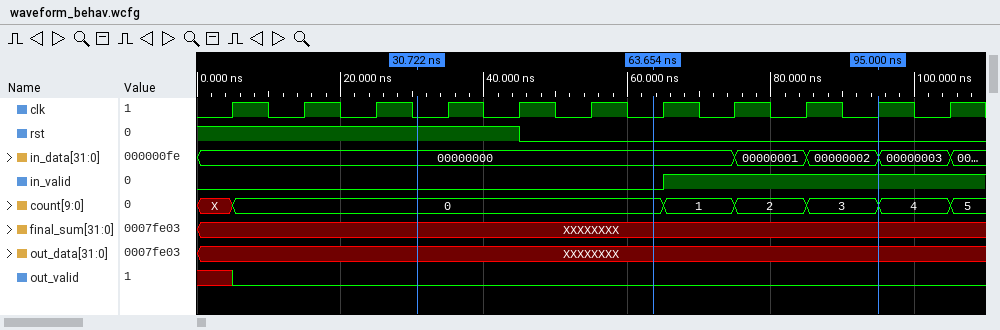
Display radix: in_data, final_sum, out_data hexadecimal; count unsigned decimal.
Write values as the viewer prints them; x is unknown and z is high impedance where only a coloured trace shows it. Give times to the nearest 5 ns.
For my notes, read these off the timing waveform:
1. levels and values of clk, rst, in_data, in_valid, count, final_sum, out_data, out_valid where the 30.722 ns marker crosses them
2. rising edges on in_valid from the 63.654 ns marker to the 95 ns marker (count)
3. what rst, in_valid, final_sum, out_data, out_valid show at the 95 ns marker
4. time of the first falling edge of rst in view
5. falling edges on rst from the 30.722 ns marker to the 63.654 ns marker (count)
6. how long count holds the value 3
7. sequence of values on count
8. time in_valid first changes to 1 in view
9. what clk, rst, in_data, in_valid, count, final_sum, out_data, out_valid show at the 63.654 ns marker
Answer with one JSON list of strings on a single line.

["clk=0, rst=1, in_data=00000000, in_valid=0, count=0, final_sum=XXXXXXXX, out_data=XXXXXXXX, out_valid=0", "1", "rst=0, in_valid=1, final_sum=XXXXXXXX, out_data=XXXXXXXX, out_valid=0", "45 ns", "1", "10 ns", "X, 0, 1, 2, 3, 4, 5", "65 ns", "clk=0, rst=0, in_data=00000000, in_valid=0, count=0, final_sum=XXXXXXXX, out_data=XXXXXXXX, out_valid=0"]
